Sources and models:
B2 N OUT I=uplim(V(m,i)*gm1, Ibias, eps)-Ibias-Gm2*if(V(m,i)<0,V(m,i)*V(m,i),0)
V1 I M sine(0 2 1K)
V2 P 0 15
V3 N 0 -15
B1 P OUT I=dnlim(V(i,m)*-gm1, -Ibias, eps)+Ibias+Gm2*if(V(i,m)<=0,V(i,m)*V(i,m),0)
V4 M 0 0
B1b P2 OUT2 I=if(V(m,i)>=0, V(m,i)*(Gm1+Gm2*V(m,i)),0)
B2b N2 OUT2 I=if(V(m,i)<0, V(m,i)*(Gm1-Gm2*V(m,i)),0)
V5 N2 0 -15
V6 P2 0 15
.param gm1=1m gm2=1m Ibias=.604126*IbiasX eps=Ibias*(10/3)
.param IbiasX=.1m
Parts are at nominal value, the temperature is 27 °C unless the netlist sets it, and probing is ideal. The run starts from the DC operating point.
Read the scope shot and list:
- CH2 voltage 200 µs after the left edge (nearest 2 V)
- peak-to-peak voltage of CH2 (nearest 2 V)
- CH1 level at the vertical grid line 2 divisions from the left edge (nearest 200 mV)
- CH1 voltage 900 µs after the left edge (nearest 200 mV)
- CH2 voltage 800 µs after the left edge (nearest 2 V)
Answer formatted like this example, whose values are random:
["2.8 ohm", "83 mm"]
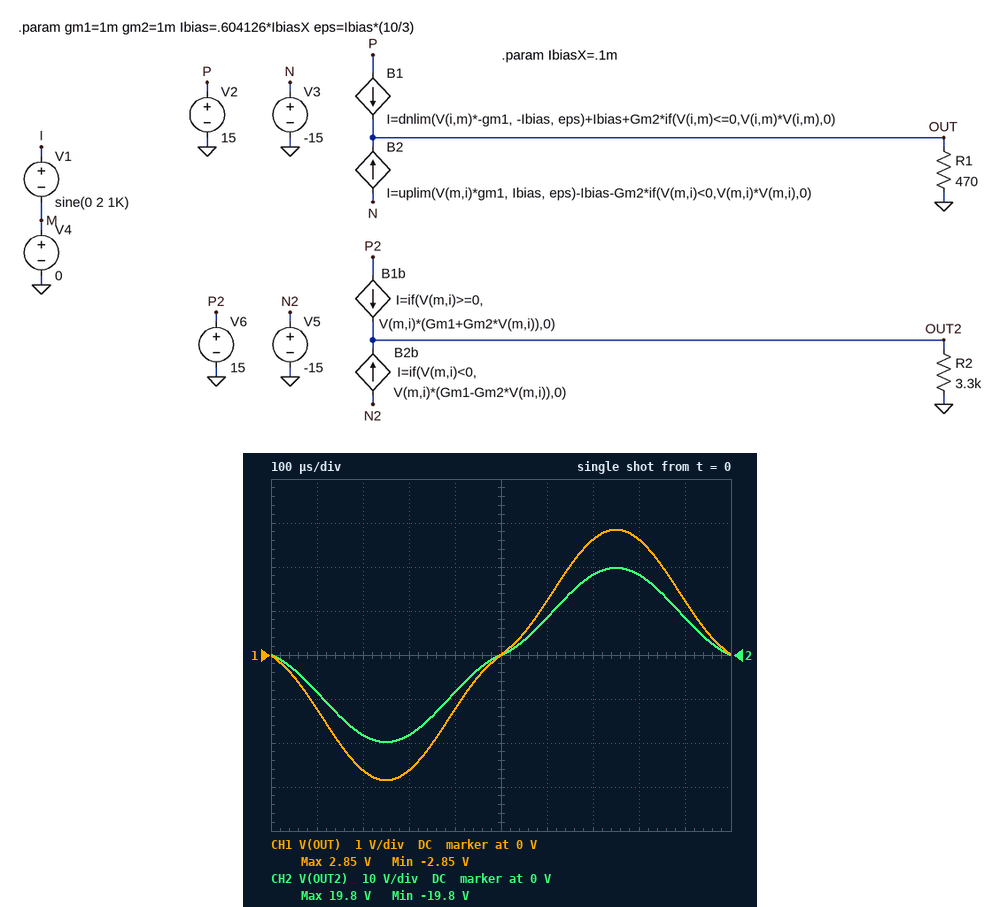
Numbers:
["-18 V", "40 V", "-2.6 V", "1.2 V", "18 V"]
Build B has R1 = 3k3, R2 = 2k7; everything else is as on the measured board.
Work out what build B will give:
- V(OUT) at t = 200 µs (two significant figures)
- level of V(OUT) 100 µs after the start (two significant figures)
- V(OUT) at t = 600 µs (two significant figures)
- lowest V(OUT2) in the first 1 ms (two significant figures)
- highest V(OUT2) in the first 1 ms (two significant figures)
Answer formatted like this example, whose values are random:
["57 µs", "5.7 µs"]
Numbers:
["-18 V", "-8.6 V", "8.6 V", "-16 V", "16 V"]
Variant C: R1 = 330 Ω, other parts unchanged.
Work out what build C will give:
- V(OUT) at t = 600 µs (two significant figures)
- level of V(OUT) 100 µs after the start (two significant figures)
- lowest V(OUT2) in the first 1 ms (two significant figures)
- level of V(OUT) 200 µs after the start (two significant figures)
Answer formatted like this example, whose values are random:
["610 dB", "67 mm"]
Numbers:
["860 mV", "-860 mV", "-20 V", "-1.8 V"]
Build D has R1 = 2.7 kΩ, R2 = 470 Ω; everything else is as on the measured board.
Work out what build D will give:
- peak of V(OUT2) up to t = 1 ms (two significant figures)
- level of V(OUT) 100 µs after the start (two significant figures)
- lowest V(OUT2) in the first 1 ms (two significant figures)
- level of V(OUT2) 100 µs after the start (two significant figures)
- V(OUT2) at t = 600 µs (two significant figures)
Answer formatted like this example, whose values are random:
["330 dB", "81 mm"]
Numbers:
["2.8 V", "-7.1 V", "-2.8 V", "-1.2 V", "1.2 V"]
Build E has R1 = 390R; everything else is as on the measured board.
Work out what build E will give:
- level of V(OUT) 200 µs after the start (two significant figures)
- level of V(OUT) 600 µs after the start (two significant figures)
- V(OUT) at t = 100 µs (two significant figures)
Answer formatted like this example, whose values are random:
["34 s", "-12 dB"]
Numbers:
["-2.2 V", "1.0 V", "-1.0 V"]
